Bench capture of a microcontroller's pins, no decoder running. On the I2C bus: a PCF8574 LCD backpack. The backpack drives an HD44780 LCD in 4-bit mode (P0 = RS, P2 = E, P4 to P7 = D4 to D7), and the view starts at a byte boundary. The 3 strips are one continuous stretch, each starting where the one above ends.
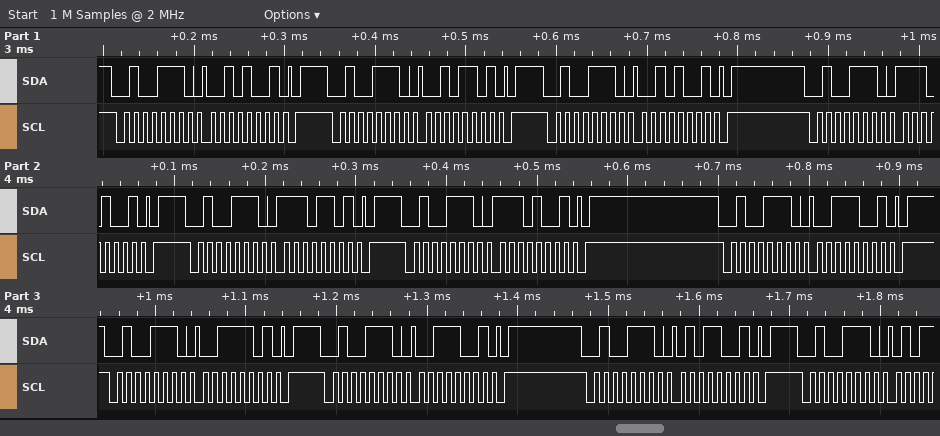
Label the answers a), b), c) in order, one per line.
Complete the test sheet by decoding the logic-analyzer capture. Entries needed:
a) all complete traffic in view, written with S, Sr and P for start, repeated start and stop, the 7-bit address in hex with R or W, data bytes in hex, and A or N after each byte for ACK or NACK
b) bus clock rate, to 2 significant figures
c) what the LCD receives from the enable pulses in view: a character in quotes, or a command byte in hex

a) S 27W A 29 A P S 27W A 2D A P S 27W A 29 A P S 27W A E9 A P S 27W A ED A P S 27W A E9 A P S 27W A 39 A P S 27W A 3D A P S 27W A 39 A P S 27W A 59 A P S 27W A
b) 100 kHz
c) '.'
